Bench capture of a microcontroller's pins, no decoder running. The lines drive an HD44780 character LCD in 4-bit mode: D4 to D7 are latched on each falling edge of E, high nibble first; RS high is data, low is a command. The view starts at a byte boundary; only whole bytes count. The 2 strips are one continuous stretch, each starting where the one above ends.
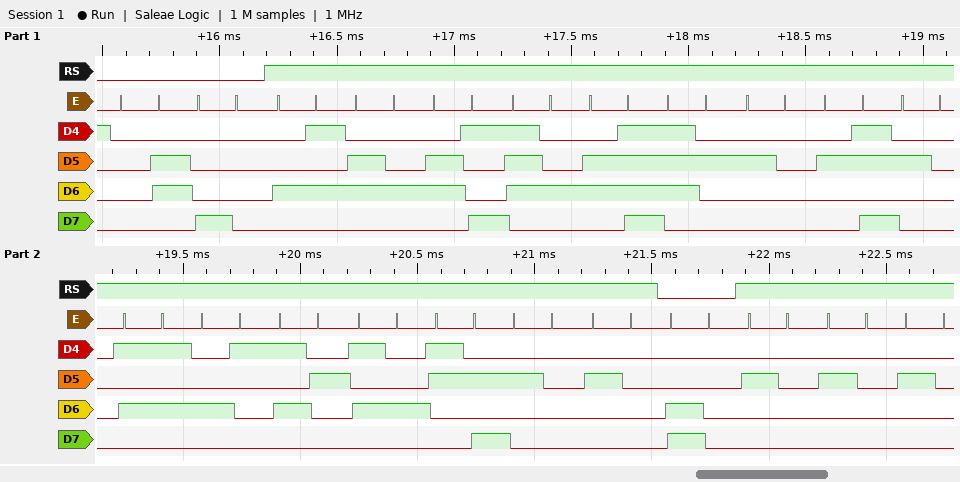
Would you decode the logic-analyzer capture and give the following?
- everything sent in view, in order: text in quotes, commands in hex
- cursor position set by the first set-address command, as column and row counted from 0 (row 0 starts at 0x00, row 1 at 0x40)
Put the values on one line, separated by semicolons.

0x06 0x80 "Editor + UART:  " 0xC0 "   "; column 0, row 0
